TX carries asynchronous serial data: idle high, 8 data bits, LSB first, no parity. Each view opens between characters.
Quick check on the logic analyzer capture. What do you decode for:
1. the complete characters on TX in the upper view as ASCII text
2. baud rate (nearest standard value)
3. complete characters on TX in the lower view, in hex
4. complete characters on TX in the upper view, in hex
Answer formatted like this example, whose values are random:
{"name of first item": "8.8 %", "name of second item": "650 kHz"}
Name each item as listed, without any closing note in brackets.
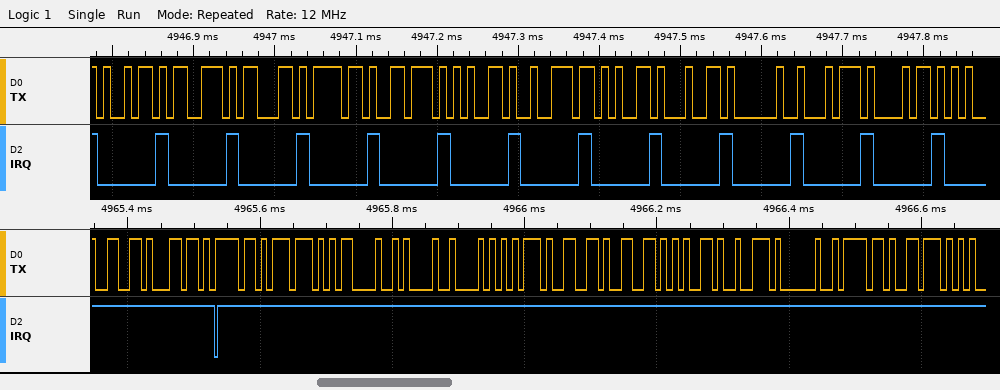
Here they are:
{"the complete characters on TX in the upper view as ASCII text": "\"iscovered th\"", "baud rate": "115200 baud", "complete characters on TX in the lower view, in hex": "66, 6C, 6F, 77, 0D, 0A, 42, 75, 66, 66, 65, 72, 20, 6F, 76", "complete characters on TX in the upper view, in hex": "69, 73, 63, 6F, 76, 65, 72, 65, 64, 20, 74, 68"}
